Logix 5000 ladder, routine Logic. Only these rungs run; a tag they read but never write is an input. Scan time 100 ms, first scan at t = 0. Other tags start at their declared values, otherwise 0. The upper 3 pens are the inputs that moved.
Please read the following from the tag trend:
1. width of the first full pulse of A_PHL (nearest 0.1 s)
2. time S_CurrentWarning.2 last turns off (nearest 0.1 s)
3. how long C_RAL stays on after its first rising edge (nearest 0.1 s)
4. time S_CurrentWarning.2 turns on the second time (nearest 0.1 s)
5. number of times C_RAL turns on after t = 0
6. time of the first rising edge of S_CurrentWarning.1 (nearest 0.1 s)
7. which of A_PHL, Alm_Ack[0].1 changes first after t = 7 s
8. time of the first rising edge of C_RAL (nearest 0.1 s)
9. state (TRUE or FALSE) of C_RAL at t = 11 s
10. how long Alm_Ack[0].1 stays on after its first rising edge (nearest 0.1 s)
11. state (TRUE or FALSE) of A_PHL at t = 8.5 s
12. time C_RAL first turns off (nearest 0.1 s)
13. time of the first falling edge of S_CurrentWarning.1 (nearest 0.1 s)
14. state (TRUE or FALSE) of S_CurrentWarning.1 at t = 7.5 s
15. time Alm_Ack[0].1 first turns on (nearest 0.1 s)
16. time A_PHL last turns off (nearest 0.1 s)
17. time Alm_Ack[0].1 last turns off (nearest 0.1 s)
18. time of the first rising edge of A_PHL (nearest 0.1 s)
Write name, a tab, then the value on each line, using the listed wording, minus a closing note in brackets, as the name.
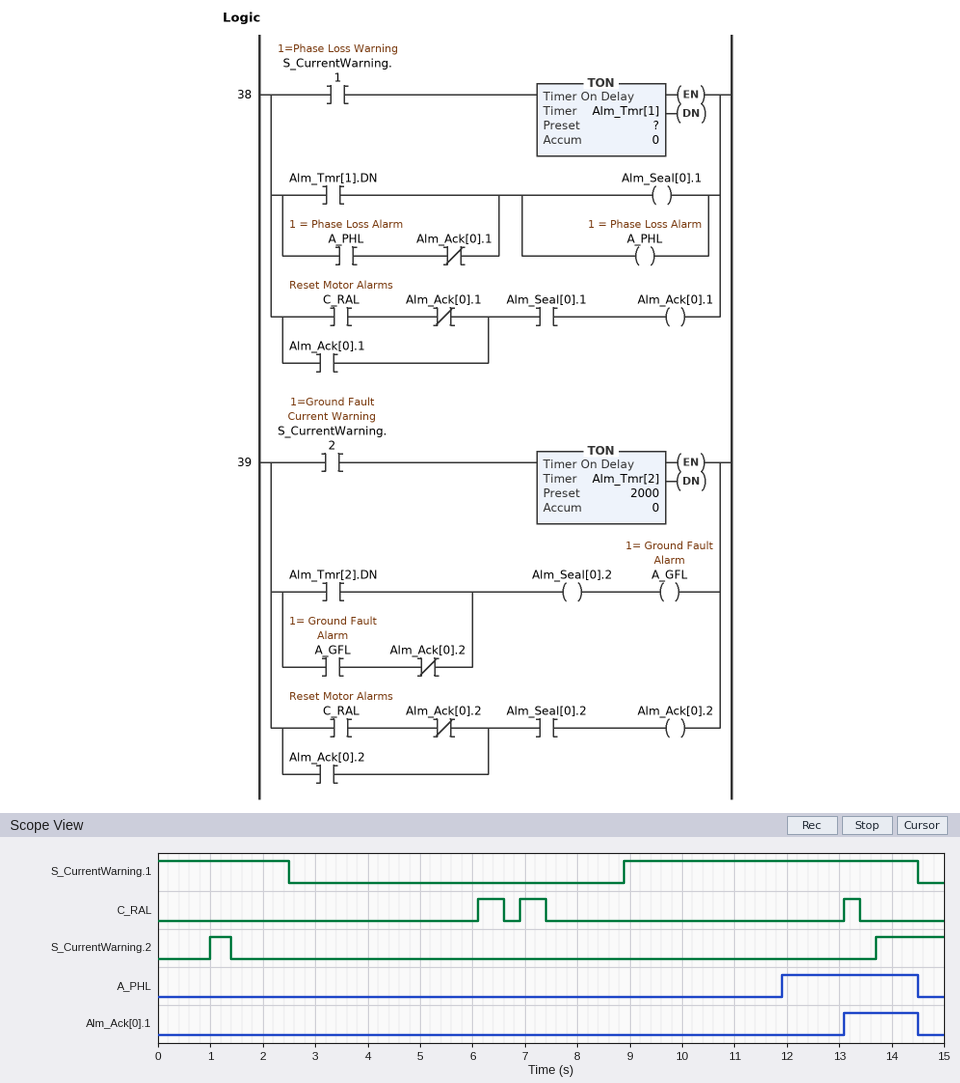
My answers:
width of the first full pulse of A_PHL	2.6 s
time S_CurrentWarning.2 last turns off	1.4 s
how long C_RAL stays on after its first rising edge	0.5 s
time S_CurrentWarning.2 turns on the second time	13.7 s
number of times C_RAL turns on after t = 0	3
time of the first rising edge of S_CurrentWarning.1	8.9 s
which of A_PHL, Alm_Ack[0].1 changes first after t = 7 s	A_PHL
time of the first rising edge of C_RAL	6.1 s
state (TRUE or FALSE) of C_RAL at t = 11 s	FALSE
how long Alm_Ack[0].1 stays on after its first rising edge	1.4 s
state (TRUE or FALSE) of A_PHL at t = 8.5 s	FALSE
time C_RAL first turns off	6.6 s
time of the first falling edge of S_CurrentWarning.1	2.5 s
state (TRUE or FALSE) of S_CurrentWarning.1 at t = 7.5 s	FALSE
time Alm_Ack[0].1 first turns on	13.1 s
time A_PHL last turns off	14.5 s
time Alm_Ack[0].1 last turns off	14.5 s
time of the first rising edge of A_PHL	11.9 s
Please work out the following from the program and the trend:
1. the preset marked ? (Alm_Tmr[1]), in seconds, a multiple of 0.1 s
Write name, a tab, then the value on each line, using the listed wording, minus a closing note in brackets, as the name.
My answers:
the preset marked ? (Alm_Tmr[1]), in seconds, a multiple of 0.1 s	3.0 s
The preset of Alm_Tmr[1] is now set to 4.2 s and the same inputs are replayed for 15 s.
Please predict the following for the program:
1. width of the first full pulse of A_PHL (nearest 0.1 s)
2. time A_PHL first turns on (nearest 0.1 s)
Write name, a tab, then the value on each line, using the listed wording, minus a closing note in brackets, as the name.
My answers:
width of the first full pulse of A_PHL	1.4 s
time A_PHL first turns on	13.1 s
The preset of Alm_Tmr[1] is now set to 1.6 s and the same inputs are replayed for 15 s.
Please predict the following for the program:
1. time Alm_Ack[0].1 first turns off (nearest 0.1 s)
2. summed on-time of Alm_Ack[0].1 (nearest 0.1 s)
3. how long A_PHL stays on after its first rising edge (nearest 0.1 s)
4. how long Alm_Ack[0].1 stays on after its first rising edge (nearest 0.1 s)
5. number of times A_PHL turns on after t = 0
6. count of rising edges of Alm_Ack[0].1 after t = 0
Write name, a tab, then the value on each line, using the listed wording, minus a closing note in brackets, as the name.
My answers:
time Alm_Ack[0].1 first turns off	6.2 s
summed on-time of Alm_Ack[0].1	1.5 s
how long A_PHL stays on after its first rising edge	4.6 s
how long Alm_Ack[0].1 stays on after its first rising edge	0.1 s
number of times A_PHL turns on after t = 0	2
count of rising edges of Alm_Ack[0].1 after t = 0	2
